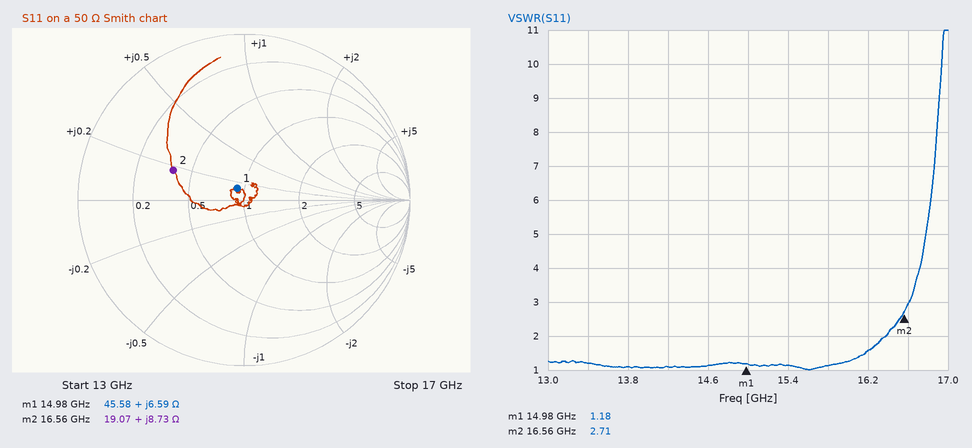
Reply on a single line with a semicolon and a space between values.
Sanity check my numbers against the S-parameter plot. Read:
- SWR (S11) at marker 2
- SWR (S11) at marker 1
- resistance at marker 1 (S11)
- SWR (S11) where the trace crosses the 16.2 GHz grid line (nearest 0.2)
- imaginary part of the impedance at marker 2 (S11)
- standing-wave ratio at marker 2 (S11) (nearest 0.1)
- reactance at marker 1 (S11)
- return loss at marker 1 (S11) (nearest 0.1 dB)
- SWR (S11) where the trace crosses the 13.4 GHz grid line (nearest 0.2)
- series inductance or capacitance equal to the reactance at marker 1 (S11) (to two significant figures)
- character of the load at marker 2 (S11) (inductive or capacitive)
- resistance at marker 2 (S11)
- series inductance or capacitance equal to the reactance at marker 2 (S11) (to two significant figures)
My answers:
2.71; 1.18; 45.58 Ω; 1.6; +8.73 Ω; 2.7; +6.59 Ω; 21.6 dB; 1.2; 70 pH; inductive; 19.07 Ω; 84 pH
